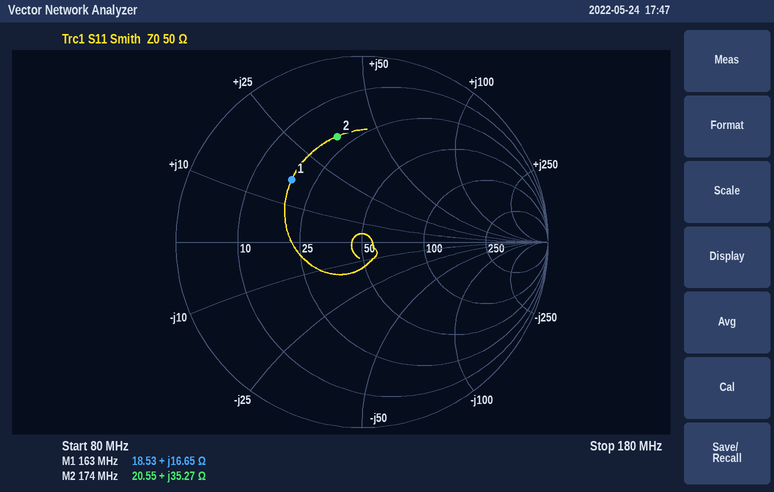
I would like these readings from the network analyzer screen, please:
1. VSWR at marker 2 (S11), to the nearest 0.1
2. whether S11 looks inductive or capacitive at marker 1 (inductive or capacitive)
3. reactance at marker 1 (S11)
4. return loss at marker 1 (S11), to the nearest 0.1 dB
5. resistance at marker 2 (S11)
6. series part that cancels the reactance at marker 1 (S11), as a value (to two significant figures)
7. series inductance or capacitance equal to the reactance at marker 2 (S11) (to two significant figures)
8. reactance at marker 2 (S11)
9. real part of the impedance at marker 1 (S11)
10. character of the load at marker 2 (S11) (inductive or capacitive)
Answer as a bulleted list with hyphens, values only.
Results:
- 3.8
- inductive
- +16.65 Ω
- 5.9 dB
- 20.55 Ω
- 59 pF
- 32 nH
- +35.27 Ω
- 18.53 Ω
- inductive
